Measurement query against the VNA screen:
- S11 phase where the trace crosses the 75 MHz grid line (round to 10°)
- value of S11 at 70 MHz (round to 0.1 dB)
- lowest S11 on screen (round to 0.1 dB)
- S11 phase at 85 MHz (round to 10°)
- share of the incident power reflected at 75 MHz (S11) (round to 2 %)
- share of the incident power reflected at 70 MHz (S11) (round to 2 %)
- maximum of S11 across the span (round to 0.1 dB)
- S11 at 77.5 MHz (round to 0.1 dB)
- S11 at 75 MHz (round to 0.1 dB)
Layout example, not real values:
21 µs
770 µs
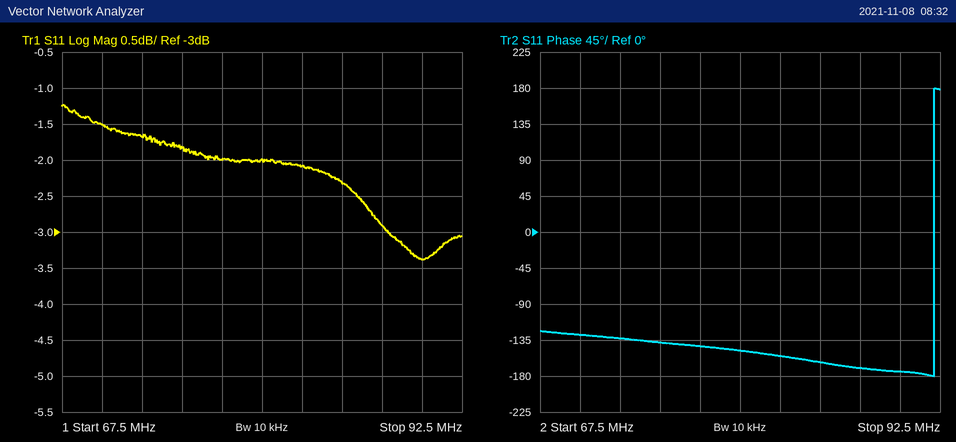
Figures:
-140°
-1.5 dB
-3.4 dB
-160°
66 %
70 %
-1.2 dB
-2.0 dB
-1.8 dB
